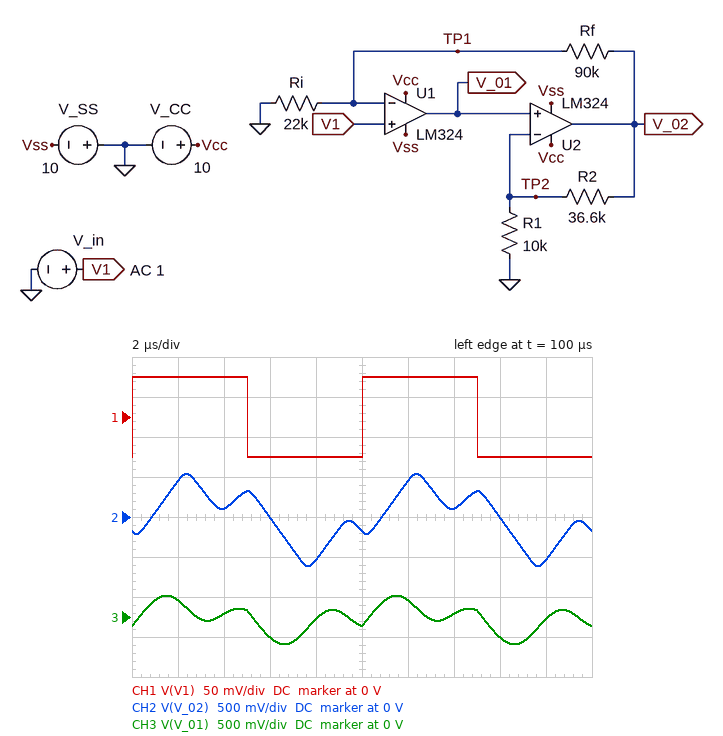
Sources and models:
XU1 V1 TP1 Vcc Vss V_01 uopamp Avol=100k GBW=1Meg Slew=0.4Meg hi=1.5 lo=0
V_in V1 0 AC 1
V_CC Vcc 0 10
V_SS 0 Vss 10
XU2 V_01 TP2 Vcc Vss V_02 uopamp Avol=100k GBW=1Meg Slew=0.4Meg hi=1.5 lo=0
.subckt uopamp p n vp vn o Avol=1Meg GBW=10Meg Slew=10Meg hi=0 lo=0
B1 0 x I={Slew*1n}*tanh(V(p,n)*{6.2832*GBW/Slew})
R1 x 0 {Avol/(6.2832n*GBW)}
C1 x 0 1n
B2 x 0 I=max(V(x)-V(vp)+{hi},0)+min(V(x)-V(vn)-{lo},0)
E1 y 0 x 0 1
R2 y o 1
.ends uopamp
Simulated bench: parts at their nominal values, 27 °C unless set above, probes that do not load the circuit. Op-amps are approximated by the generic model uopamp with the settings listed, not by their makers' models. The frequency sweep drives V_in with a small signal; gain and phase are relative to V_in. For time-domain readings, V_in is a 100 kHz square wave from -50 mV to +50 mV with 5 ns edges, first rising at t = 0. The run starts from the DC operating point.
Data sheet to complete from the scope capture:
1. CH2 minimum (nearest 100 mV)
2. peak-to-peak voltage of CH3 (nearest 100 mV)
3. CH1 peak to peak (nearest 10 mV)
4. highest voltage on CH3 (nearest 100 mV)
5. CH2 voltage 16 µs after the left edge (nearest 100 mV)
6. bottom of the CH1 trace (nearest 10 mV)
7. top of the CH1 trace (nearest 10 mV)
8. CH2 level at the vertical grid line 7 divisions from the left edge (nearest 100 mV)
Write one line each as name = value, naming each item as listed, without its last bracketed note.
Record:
CH2 minimum = -600 mV
peak-to-peak voltage of CH3 = 600 mV
CH1 peak to peak = 100 mV
highest voltage on CH3 = 300 mV
CH2 voltage 16 µs after the left edge = 0 V
bottom of the CH1 trace = -50 mV
top of the CH1 trace = 50 mV
CH2 level at the vertical grid line 7 divisions from the left edge = 100 mV
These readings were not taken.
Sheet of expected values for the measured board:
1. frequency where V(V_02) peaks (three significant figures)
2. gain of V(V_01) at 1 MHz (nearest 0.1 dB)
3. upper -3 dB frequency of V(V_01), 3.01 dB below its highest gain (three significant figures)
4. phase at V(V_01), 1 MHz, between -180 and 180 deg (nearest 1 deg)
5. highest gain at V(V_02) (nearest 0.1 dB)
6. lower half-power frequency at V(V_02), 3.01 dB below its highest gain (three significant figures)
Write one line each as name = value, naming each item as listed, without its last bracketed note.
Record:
frequency where V(V_02) peaks = 416 kHz
gain of V(V_01) at 1 MHz = 1.8 dB
upper -3 dB frequency of V(V_01), 3.01 dB below its highest gain = 554 kHz
phase at V(V_01), 1 MHz, between -180 and 180 deg = -87 deg
highest gain at V(V_02) = 20.7 dB
lower half-power frequency at V(V_02), 3.01 dB below its highest gain = 285 kHz
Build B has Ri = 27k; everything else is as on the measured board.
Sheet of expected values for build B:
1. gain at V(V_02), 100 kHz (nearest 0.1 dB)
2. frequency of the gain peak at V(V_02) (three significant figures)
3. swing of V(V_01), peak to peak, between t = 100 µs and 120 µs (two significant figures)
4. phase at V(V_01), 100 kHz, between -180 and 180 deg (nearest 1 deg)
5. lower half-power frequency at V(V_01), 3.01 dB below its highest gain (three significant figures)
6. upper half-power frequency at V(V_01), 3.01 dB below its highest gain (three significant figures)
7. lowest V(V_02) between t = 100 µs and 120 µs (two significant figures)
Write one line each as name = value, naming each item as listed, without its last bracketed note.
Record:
gain at V(V_02), 100 kHz = 13.1 dB
frequency of the gain peak at V(V_02) = 456 kHz
swing of V(V_01), peak to peak, between t = 100 µs and 120 µs = 620 mV
phase at V(V_01), 100 kHz, between -180 and 180 deg = 19 deg
lower half-power frequency at V(V_01), 3.01 dB below its highest gain = 377 kHz
upper half-power frequency at V(V_01), 3.01 dB below its highest gain = 592 kHz
lowest V(V_02) between t = 100 µs and 120 µs = -540 mV
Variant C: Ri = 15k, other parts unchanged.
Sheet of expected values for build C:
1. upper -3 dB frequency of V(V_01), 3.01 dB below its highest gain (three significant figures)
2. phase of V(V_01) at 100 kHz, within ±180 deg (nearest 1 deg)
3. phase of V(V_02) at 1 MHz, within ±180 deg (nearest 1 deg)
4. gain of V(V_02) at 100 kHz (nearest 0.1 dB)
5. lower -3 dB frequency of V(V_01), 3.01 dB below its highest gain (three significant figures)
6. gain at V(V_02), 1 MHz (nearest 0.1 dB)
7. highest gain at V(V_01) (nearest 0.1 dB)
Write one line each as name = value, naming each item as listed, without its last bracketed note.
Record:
upper -3 dB frequency of V(V_01), 3.01 dB below its highest gain = 486 kHz
phase of V(V_01) at 100 kHz, within ±180 deg = 16 deg
phase of V(V_02) at 1 MHz, within ±180 deg = -166 deg
gain of V(V_02) at 100 kHz = 17.4 dB
lower -3 dB frequency of V(V_01), 3.01 dB below its highest gain = 270 kHz
gain at V(V_02), 1 MHz = 1.1 dB
highest gain at V(V_01) = 14.6 dB
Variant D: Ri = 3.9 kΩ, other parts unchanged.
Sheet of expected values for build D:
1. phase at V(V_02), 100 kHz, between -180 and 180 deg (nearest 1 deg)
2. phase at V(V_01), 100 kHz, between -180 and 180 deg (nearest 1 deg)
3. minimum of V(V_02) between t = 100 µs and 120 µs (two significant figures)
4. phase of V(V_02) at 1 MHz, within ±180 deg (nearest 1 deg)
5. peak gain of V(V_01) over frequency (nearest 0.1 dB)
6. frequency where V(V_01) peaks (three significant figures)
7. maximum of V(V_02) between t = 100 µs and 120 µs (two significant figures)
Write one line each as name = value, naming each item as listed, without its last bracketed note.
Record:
phase at V(V_02), 100 kHz, between -180 and 180 deg = -34 deg
phase at V(V_01), 100 kHz, between -180 and 180 deg = -9 deg
minimum of V(V_02) between t = 100 µs and 120 µs = -950 mV
phase of V(V_02) at 1 MHz, within ±180 deg = -167 deg
peak gain of V(V_01) over frequency = 17.0 dB
frequency where V(V_01) peaks = 169 kHz
maximum of V(V_02) between t = 100 µs and 120 µs = 950 mV
